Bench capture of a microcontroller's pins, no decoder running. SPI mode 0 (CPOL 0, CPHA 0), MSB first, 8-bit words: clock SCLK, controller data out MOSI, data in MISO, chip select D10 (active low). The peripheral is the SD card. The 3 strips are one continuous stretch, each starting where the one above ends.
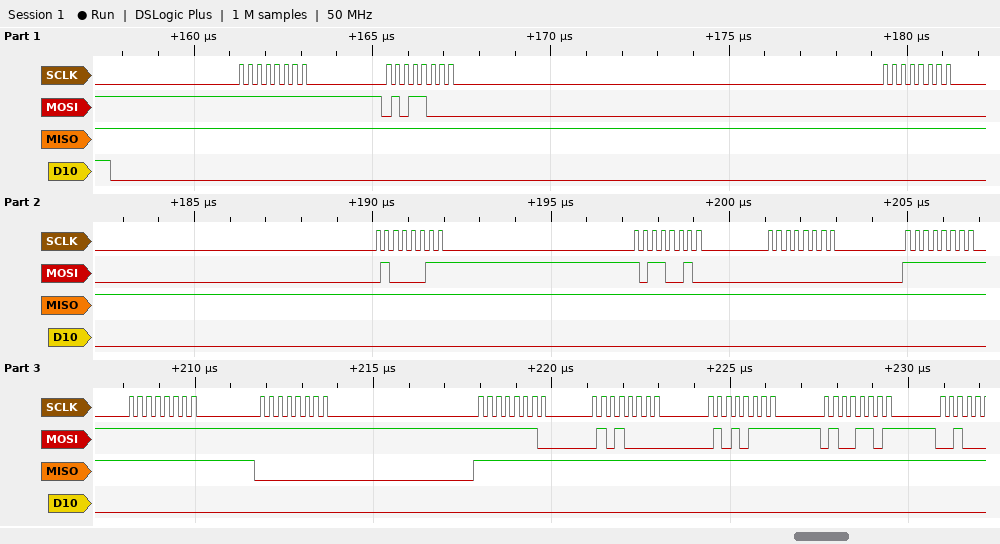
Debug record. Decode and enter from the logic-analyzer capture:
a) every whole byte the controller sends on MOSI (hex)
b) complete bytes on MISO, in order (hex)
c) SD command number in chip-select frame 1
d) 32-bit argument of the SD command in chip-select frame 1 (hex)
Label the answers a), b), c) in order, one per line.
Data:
a) FF 58 00 43 B2 00 FF FF FF FE 50 57 4D
b) FF FF FF FF FF FF FF FF 00 FF FF FF FF
c) CMD24
d) 0x0043B200
